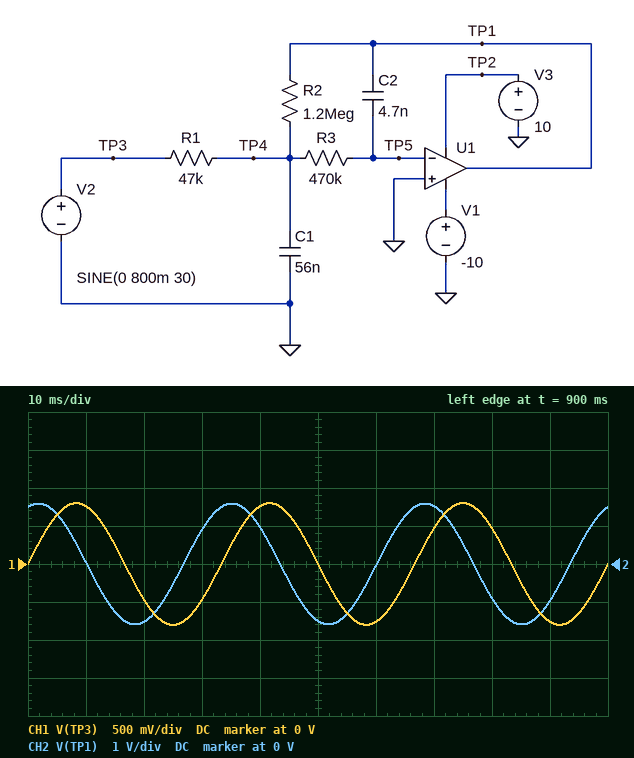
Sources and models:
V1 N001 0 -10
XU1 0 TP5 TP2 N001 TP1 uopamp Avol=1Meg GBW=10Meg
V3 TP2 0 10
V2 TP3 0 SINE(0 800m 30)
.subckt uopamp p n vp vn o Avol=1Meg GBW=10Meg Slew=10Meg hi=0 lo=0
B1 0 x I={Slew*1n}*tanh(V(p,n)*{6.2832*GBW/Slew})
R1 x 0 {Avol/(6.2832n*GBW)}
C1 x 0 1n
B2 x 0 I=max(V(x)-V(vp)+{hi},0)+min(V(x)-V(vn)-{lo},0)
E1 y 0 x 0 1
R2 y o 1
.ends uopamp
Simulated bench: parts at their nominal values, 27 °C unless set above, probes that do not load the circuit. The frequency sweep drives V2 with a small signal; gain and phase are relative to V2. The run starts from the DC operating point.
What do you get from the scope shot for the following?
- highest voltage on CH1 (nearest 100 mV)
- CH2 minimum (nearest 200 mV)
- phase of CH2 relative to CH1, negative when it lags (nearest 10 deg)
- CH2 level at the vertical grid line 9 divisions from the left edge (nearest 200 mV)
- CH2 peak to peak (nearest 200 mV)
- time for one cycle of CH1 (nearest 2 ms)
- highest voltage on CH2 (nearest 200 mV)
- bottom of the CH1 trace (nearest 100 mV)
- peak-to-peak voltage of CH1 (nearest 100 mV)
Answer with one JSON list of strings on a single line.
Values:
["800 mV", "-1.6 V", "70 deg", "-1.0 V", "3.2 V", "34 ms", "1.6 V", "-800 mV", "1.6 V"]
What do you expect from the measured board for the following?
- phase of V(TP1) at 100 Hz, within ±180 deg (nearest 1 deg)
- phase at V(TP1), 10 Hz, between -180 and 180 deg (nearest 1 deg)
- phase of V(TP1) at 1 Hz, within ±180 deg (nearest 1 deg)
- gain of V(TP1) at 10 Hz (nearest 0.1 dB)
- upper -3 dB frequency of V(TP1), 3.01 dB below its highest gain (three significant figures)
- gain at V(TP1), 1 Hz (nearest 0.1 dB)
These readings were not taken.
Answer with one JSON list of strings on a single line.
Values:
["35 deg", "96 deg", "158 deg", "16.0 dB", "2.57 Hz", "27.5 dB"]
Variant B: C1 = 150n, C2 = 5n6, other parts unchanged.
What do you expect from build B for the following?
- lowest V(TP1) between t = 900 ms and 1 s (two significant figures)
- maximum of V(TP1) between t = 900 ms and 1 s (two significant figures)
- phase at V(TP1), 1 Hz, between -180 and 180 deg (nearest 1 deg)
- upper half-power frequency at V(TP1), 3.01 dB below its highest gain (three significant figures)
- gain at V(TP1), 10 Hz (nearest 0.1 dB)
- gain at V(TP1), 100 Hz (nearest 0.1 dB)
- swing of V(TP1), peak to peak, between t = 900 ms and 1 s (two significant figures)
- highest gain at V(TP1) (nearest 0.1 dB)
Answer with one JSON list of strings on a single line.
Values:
["-950 mV", "950 mV", "154 deg", "2.26 Hz", "14.4 dB", "-17.5 dB", "1.9 V", "28.1 dB"]
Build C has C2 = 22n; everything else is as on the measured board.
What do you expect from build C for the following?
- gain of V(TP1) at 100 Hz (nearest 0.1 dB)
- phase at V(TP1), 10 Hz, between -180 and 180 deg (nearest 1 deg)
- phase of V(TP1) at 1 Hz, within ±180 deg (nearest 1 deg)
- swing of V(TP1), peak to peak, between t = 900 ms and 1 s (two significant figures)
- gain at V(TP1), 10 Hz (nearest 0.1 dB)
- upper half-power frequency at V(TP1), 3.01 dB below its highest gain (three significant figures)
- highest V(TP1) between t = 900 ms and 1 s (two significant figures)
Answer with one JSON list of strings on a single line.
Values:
["-22.3 dB", "85 deg", "117 deg", "670 mV", "2.6 dB", "533 mHz", "320 mV"]
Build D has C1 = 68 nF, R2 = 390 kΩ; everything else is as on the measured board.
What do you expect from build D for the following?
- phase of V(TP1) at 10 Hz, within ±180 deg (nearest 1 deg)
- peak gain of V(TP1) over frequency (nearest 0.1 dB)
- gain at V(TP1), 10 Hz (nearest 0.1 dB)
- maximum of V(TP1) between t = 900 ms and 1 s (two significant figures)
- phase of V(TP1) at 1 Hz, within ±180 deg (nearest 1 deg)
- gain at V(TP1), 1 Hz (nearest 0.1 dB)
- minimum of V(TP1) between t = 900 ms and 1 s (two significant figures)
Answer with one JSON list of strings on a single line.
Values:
["119 deg", "18.4 dB", "14.3 dB", "1.5 V", "172 deg", "18.3 dB", "-1.5 V"]
